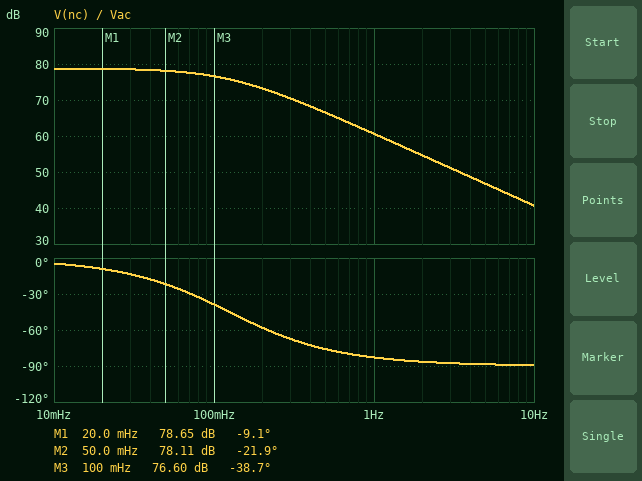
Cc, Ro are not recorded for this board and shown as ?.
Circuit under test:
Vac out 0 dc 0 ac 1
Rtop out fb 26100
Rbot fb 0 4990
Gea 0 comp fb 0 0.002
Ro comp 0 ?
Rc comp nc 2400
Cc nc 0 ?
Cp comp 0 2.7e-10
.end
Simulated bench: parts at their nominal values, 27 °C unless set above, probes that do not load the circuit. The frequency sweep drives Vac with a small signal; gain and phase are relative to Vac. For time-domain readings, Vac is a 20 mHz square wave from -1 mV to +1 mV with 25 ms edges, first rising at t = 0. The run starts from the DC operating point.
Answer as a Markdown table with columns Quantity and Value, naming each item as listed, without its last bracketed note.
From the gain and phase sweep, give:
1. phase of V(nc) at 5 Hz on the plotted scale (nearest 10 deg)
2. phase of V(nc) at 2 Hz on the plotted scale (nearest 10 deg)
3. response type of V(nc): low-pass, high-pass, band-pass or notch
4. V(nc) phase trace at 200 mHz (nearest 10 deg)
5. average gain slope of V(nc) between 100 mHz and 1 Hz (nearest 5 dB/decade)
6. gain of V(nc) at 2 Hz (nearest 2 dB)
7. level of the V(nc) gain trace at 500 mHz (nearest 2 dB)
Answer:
| Quantity | Value |
|---|---|
| phase of V(nc) at 5 Hz on the plotted scale | -90 deg |
| phase of V(nc) at 2 Hz on the plotted scale | -90 deg |
| response type of V(nc): low-pass, high-pass, band-pass or notch | low-pass |
| V(nc) phase trace at 200 mHz | -60 deg |
| average gain slope of V(nc) between 100 mHz and 1 Hz | -15 dB/decade |
| gain of V(nc) at 2 Hz | 54 dB |
| level of the V(nc) gain trace at 500 mHz | 66 dB |
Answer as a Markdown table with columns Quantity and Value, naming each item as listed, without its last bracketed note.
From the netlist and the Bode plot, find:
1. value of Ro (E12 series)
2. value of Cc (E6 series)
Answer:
| Quantity | Value |
|---|---|
| value of Ro | 27 MΩ |
| value of Cc | 47 nF |
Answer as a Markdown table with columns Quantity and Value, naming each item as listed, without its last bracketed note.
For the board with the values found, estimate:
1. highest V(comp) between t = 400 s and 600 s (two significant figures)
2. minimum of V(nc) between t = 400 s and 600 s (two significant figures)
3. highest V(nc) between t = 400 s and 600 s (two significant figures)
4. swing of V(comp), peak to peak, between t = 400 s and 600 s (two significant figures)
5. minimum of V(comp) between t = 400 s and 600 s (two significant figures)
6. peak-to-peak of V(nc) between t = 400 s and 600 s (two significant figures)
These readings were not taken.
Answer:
| Quantity | Value |
|---|---|
| highest V(comp) between t = 400 s and 600 s | 8.7 V |
| minimum of V(nc) between t = 400 s and 600 s | -8.7 V |
| highest V(nc) between t = 400 s and 600 s | 8.7 V |
| swing of V(comp), peak to peak, between t = 400 s and 600 s | 17 V |
| minimum of V(comp) between t = 400 s and 600 s | -8.7 V |
| peak-to-peak of V(nc) between t = 400 s and 600 s | 17 V |
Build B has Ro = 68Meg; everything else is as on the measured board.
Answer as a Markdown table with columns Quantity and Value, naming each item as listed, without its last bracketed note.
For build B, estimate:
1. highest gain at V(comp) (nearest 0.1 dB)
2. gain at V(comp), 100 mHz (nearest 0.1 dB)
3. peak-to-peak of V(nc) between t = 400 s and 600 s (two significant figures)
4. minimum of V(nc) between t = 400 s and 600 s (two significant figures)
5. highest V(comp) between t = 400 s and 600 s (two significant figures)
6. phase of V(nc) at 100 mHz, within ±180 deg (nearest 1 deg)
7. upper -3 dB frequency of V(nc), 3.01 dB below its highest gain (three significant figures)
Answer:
| Quantity | Value |
|---|---|
| highest gain at V(comp) | 86.8 dB |
| gain at V(comp), 100 mHz | 79.7 dB |
| peak-to-peak of V(nc) between t = 400 s and 600 s | 44 V |
| minimum of V(nc) between t = 400 s and 600 s | -22 V |
| highest V(comp) between t = 400 s and 600 s | 22 V |
| phase of V(nc) at 100 mHz, within ±180 deg | -64 deg |
| upper -3 dB frequency of V(nc), 3.01 dB below its highest gain | 49.5 mHz |
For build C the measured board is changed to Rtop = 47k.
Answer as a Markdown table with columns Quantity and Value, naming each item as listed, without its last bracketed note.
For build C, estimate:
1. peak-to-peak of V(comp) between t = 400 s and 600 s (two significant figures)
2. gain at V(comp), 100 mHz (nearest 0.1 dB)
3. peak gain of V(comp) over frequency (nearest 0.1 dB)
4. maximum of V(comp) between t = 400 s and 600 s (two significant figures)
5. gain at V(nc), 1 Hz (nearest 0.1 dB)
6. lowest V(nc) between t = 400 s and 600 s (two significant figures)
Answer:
| Quantity | Value |
|---|---|
| peak-to-peak of V(comp) between t = 400 s and 600 s | 10 V |
| gain at V(comp), 100 mHz | 72.1 dB |
| peak gain of V(comp) over frequency | 74.3 dB |
| maximum of V(comp) between t = 400 s and 600 s | 5.2 V |
| gain at V(nc), 1 Hz | 56.1 dB |
| lowest V(nc) between t = 400 s and 600 s | -5.2 V |
